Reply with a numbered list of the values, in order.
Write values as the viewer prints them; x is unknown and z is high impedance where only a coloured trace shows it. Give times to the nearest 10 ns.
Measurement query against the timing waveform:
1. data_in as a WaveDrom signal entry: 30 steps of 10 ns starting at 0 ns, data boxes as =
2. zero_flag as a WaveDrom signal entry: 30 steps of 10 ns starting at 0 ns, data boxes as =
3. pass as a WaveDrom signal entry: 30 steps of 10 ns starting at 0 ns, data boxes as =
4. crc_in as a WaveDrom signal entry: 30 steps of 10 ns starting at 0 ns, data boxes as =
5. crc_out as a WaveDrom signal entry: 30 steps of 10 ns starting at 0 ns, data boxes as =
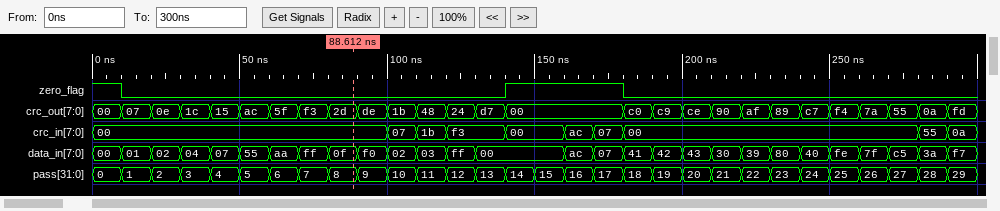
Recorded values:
1. {name: 'data_in', wave: '==============..==============', data: '00 01 02 04 07 55 aa ff 0f f0 02 03 ff 00 ac 07 41 42 43 30 39 80 40 fe 7f c5 3a f7'}
2. {name: 'zero_flag', wave: '10............1...0...........'}
3. {name: 'pass', wave: '==============================', data: '0 1 2 3 4 5 6 7 8 9 10 11 12 13 14 15 16 17 18 19 20 21 22 23 24 25 26 27 28 29'}
4. {name: 'crc_in', wave: '=.........===.=.===.........==', data: '00 07 1b f3 00 ac 07 00 55 0a'}
5. {name: 'crc_out', wave: '===============...============', data: '00 07 0e 1c 15 ac 5f f3 2d de 1b 48 24 d7 00 c0 c9 ce 90 af 89 c7 f4 7a 55 0a fd'}
